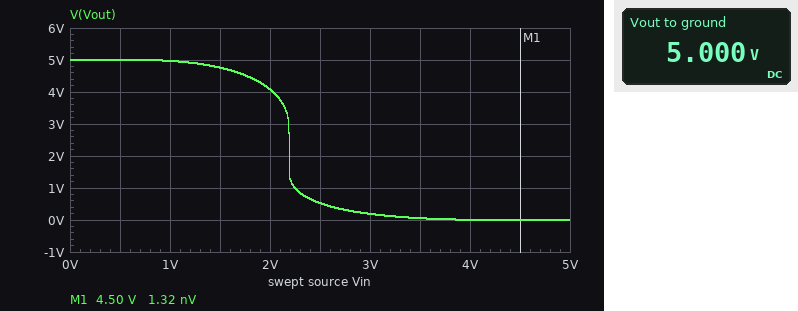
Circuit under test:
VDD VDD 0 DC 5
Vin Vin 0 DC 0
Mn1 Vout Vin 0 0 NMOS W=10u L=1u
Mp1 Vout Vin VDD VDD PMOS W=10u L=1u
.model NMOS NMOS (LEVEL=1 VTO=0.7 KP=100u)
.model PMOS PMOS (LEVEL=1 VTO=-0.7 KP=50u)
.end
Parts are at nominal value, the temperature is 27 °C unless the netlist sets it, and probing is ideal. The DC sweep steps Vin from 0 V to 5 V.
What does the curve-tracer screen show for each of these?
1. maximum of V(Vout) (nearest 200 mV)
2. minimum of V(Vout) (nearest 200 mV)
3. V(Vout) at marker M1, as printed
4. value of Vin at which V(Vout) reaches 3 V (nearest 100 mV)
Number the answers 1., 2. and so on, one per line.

1. 5.0 V
2. 0 V
3. 1.32 nV
4. 2.2 V
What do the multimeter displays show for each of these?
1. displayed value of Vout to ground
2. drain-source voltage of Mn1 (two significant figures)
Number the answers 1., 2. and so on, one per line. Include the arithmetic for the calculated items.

1. 5.000 V
2. 5 V = 5.0 V
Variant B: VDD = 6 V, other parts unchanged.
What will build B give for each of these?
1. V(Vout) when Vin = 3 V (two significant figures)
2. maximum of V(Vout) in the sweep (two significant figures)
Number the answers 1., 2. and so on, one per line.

1. 670 mV
2. 6.0 V
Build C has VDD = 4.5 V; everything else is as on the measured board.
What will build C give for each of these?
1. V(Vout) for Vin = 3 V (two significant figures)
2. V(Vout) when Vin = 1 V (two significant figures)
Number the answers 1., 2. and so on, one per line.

1. 71 mV
2. 4.5 V
